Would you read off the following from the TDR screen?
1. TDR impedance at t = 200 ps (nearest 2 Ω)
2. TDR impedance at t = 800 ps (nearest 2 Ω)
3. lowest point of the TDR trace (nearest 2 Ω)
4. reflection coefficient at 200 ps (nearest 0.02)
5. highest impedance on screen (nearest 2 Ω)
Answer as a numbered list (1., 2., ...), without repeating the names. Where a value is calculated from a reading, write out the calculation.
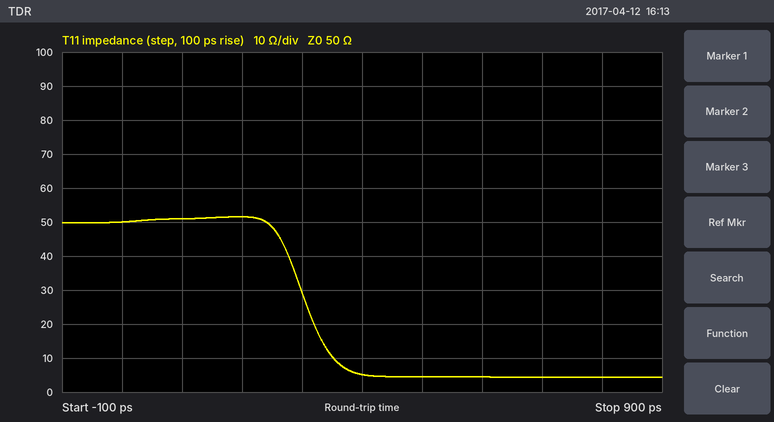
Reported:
1. 52 Ω
2. 4 Ω
3. 4 Ω
4. (52 − 50)/(52 + 50) ≈ +0.02
5. 52 Ω
